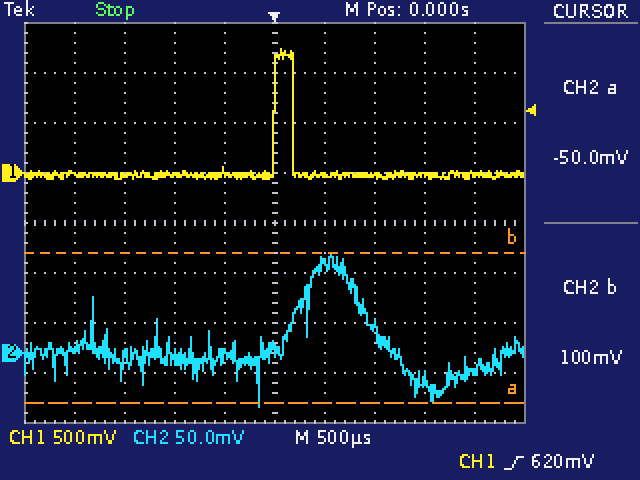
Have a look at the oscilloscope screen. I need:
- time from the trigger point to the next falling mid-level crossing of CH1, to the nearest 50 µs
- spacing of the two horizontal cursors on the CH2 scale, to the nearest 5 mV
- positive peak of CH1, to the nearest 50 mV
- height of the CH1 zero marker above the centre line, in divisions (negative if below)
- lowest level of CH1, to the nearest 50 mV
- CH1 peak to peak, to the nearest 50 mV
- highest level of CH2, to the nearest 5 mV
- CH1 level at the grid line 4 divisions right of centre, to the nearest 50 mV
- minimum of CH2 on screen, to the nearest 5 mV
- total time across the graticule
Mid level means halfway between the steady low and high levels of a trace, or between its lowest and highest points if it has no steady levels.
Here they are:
200 µs
150 mV
1.25 V
+1.0 div
-50 mV
1.30 V
100 mV
0 mV
-55 mV
5 ms
